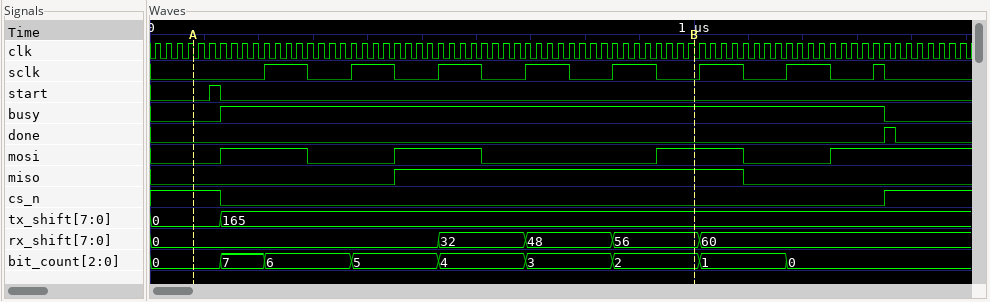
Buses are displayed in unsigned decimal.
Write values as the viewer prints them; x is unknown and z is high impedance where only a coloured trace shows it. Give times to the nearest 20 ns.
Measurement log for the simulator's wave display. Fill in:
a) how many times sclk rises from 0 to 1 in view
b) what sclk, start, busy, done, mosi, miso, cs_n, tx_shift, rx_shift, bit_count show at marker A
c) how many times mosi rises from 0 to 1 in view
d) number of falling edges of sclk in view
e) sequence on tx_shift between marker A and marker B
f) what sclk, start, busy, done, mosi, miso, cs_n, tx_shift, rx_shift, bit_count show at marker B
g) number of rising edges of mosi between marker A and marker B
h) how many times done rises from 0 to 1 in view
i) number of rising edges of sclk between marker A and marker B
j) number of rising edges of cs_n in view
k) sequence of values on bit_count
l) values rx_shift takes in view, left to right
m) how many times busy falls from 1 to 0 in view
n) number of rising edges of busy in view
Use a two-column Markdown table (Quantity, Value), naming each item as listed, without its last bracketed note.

| Quantity | Value |
|---|---|
| how many times sclk rises from 0 to 1 in view | 8 |
| what sclk, start, busy, done, mosi, miso, cs_n, tx_shift, rx_shift, bit_count show at marker A | sclk=0, start=0, busy=0, done=0, mosi=0, miso=0, cs_n=1, tx_shift=0, rx_shift=0, bit_count=0 |
| how many times mosi rises from 0 to 1 in view | 4 |
| number of falling edges of sclk in view | 8 |
| sequence on tx_shift between marker A and marker B | 0, 165 |
| what sclk, start, busy, done, mosi, miso, cs_n, tx_shift, rx_shift, bit_count show at marker B | sclk=0, start=0, busy=1, done=0, mosi=1, miso=1, cs_n=0, tx_shift=165, rx_shift=56, bit_count=2 |
| number of rising edges of mosi between marker A and marker B | 3 |
| how many times done rises from 0 to 1 in view | 1 |
| number of rising edges of sclk between marker A and marker B | 5 |
| number of rising edges of cs_n in view | 1 |
| sequence of values on bit_count | 0, 7, 6, 5, 4, 3, 2, 1, 0 |
| values rx_shift takes in view, left to right | 0, 32, 48, 56, 60 |
| how many times busy falls from 1 to 0 in view | 1 |
| number of rising edges of busy in view | 1 |
